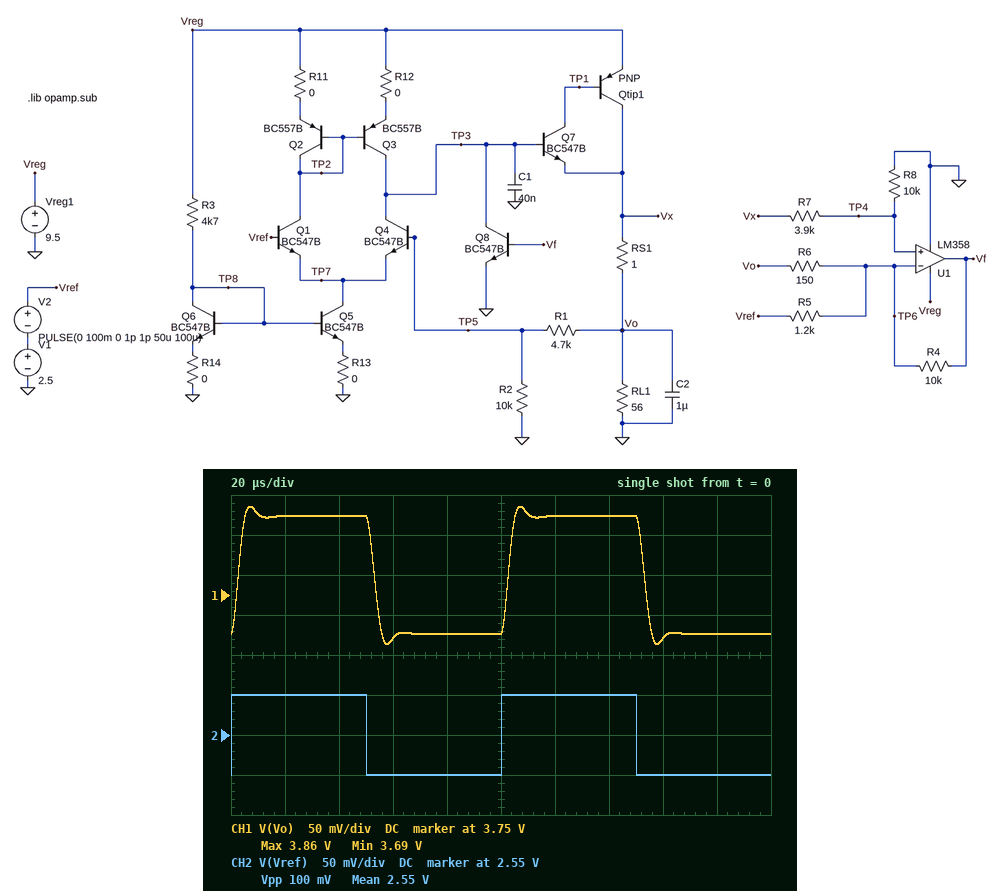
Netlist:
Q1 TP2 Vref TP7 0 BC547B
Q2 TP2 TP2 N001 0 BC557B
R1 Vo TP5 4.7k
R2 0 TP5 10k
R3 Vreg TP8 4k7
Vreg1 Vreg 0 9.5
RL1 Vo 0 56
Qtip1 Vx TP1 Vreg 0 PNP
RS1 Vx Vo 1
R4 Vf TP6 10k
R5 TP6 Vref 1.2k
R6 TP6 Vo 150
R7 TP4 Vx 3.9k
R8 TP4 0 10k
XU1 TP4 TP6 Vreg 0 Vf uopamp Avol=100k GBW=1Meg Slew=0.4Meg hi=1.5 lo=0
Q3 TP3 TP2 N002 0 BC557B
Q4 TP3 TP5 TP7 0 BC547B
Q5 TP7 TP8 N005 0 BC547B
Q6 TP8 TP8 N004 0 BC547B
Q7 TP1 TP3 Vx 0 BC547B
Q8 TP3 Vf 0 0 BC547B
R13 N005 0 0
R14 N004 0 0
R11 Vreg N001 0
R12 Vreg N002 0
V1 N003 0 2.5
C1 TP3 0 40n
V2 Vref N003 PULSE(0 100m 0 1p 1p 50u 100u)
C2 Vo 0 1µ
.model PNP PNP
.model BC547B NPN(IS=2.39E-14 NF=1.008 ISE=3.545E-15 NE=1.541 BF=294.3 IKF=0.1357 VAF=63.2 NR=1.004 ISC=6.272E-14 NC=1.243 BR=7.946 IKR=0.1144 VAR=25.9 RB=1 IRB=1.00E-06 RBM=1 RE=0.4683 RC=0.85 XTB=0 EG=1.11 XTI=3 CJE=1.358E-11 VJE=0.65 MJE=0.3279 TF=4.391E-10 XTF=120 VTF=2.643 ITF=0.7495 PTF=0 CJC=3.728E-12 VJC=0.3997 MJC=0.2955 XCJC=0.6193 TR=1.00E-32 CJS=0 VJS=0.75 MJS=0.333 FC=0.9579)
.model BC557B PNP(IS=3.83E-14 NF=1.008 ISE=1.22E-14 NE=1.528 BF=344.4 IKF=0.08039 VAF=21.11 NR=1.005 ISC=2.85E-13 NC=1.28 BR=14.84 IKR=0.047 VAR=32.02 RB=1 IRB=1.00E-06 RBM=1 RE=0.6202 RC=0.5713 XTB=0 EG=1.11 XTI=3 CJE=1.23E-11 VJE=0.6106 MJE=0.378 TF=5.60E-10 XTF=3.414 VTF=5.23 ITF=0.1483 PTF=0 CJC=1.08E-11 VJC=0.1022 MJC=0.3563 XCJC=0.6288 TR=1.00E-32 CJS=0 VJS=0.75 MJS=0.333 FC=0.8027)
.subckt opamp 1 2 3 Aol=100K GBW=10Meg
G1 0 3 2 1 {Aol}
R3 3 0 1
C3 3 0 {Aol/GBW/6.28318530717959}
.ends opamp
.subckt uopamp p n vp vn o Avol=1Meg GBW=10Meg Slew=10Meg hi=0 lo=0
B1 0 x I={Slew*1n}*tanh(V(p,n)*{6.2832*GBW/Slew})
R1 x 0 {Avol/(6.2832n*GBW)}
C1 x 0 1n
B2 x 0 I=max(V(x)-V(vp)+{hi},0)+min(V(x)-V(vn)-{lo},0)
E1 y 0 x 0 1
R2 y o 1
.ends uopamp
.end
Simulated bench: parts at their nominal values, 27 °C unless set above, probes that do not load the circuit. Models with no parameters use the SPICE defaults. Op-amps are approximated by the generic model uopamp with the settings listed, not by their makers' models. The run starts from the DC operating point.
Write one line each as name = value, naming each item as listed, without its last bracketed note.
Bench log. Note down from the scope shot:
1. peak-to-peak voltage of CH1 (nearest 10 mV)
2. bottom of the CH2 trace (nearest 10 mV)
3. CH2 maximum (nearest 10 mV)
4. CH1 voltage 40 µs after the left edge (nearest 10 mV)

peak-to-peak voltage of CH1 = 170 mV
bottom of the CH2 trace = 2.50 V
CH2 maximum = 2.60 V
CH1 voltage 40 µs after the left edge = 3.85 V
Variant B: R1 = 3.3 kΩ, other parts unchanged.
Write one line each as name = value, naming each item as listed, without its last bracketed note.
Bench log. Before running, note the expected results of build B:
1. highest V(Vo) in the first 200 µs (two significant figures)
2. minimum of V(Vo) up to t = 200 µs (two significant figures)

highest V(Vo) in the first 200 µs = 3.5 V
minimum of V(Vo) up to t = 200 µs = 3.3 V
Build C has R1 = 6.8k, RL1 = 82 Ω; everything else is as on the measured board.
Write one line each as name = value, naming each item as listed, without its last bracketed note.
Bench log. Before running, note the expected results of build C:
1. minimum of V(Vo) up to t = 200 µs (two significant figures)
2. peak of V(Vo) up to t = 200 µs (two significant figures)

minimum of V(Vo) up to t = 200 µs = 4.2 V
peak of V(Vo) up to t = 200 µs = 4.4 V
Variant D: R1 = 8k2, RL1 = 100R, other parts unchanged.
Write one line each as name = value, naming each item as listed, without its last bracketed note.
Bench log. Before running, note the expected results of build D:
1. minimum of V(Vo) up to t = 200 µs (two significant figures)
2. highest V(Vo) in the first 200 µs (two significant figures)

minimum of V(Vo) up to t = 200 µs = 4.6 V
highest V(Vo) in the first 200 µs = 4.8 V
